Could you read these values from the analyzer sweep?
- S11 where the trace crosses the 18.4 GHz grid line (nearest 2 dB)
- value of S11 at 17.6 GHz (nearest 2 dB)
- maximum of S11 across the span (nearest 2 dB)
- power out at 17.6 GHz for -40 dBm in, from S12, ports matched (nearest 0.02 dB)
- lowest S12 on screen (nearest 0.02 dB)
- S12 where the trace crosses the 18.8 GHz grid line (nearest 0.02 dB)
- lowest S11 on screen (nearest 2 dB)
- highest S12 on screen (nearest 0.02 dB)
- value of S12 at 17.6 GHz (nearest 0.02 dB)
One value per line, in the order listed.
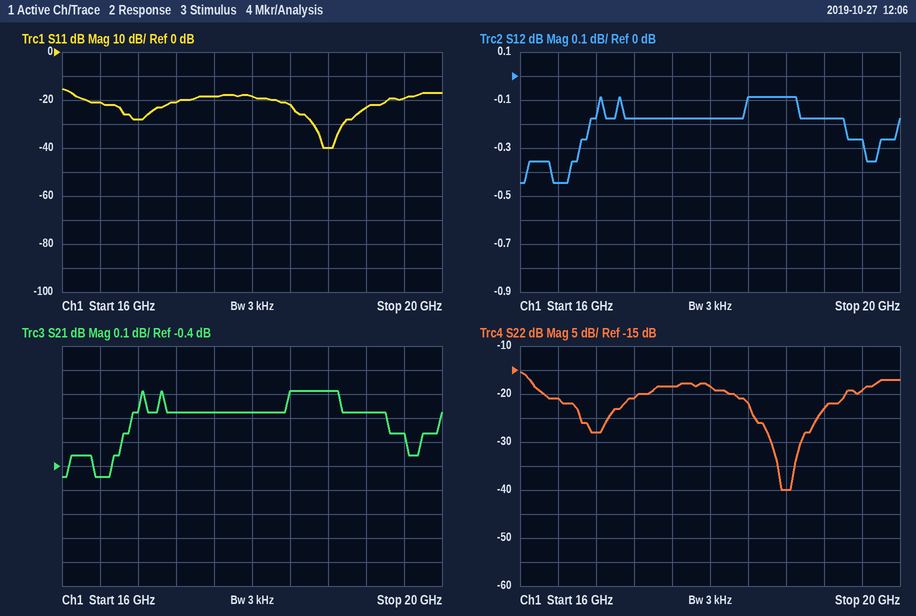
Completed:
-22 dB
-18 dB
-16 dB
-40.18 dBm
-0.44 dB
-0.08 dB
-40 dB
-0.08 dB
-0.18 dB
